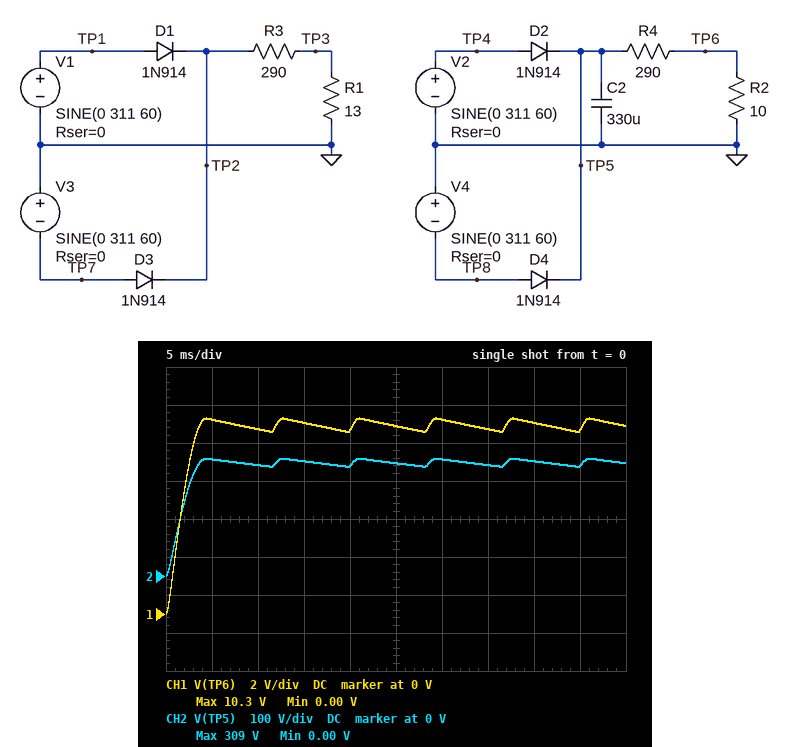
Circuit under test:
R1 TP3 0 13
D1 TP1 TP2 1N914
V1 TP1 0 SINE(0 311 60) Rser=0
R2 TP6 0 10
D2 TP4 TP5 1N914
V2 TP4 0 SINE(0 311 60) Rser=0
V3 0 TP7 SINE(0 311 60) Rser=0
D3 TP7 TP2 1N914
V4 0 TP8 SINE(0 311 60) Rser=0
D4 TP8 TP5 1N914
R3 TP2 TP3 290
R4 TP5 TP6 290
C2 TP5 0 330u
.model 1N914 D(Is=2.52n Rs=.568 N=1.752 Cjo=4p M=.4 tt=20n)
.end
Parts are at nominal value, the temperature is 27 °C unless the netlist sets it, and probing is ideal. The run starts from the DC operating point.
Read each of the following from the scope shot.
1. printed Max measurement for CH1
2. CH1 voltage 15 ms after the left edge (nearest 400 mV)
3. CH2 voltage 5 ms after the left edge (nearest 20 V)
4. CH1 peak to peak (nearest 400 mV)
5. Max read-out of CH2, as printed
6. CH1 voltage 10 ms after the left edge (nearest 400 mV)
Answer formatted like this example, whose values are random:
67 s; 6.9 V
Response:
10.3 V; 10.0 V; 300 V; 10.4 V; 309 V; 9.6 V
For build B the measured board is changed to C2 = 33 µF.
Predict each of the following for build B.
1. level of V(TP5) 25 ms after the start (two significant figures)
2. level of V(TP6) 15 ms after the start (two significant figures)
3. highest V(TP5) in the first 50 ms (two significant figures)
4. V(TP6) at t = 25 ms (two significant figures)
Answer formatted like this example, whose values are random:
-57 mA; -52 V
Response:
210 V; 8.3 V; 310 V; 7.0 V
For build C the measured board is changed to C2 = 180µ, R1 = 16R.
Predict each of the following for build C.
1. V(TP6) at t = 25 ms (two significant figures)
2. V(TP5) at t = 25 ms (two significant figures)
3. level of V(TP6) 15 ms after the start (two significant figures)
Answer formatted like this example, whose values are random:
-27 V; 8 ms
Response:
9.6 V; 290 V; 9.9 V
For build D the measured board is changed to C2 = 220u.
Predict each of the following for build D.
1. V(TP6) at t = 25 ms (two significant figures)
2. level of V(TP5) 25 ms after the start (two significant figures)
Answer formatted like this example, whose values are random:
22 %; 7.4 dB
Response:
9.7 V; 290 V
